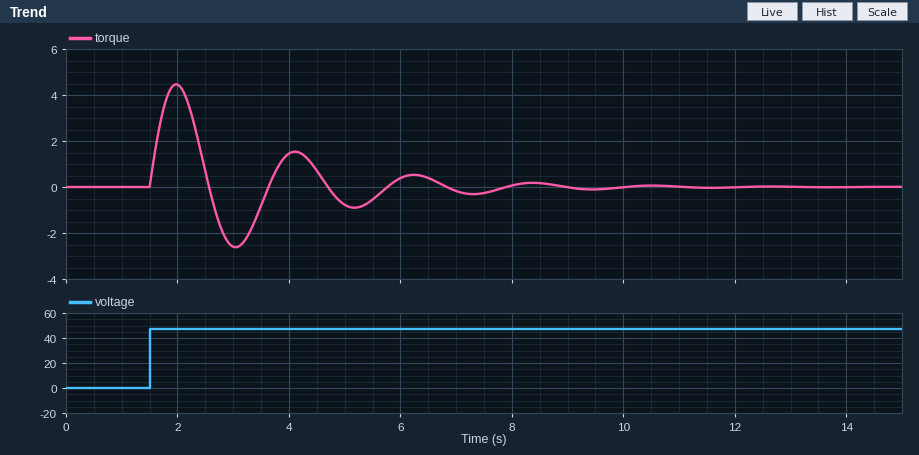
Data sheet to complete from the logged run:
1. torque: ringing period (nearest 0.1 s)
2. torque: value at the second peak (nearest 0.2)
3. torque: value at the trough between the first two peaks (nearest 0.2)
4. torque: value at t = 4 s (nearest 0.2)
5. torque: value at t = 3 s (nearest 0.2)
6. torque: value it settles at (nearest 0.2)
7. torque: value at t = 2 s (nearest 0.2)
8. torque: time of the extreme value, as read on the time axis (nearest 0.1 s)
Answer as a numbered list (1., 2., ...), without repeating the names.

1. 2.1 s
2. 1.6
3. -2.6
4. 1.4
5. -2.6
6. 0.0
7. 4.4
8. 2.0 s
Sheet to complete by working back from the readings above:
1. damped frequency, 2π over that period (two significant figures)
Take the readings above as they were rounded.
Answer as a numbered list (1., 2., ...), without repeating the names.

1. 3.0 rad/s
